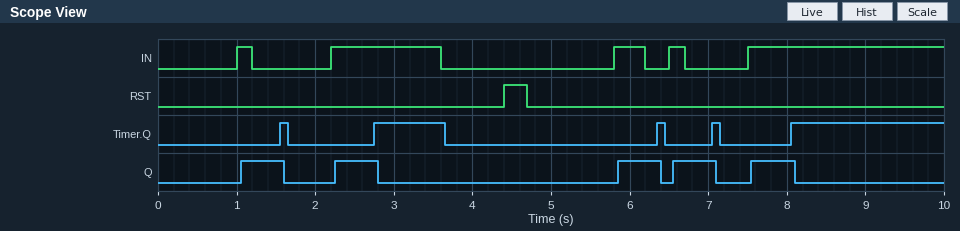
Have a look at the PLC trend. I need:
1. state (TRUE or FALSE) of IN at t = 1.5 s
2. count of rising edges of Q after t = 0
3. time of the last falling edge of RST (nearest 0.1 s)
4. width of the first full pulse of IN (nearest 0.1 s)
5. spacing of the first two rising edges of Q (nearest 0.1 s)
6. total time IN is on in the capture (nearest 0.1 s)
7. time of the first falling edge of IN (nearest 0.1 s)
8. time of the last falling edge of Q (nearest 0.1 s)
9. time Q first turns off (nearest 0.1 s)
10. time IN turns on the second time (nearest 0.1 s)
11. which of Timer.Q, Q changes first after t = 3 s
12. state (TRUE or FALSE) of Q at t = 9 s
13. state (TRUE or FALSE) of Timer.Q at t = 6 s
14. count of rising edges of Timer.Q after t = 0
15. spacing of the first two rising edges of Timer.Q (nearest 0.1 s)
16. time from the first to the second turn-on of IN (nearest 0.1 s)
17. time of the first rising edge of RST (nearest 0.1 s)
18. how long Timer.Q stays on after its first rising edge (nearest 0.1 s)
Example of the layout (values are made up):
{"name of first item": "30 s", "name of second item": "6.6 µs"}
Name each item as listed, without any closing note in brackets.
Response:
{"state (TRUE or FALSE) of IN at t = 1.5 s": "FALSE", "count of rising edges of Q after t = 0": "5", "time of the last falling edge of RST": "4.7 s", "width of the first full pulse of IN": "0.2 s", "spacing of the first two rising edges of Q": "1.2 s", "total time IN is on in the capture": "4.7 s", "time of the first falling edge of IN": "1.2 s", "time of the last falling edge of Q": "8.1 s", "time Q first turns off": "1.6 s", "time IN turns on the second time": "2.2 s", "which of Timer.Q, Q changes first after t = 3 s": "Timer.Q", "state (TRUE or FALSE) of Q at t = 9 s": "FALSE", "state (TRUE or FALSE) of Timer.Q at t = 6 s": "FALSE", "count of rising edges of Timer.Q after t = 0": "5", "spacing of the first two rising edges of Timer.Q": "1.2 s", "time from the first to the second turn-on of IN": "1.2 s", "time of the first rising edge of RST": "4.4 s", "how long Timer.Q stays on after its first rising edge": "0.1 s"}
